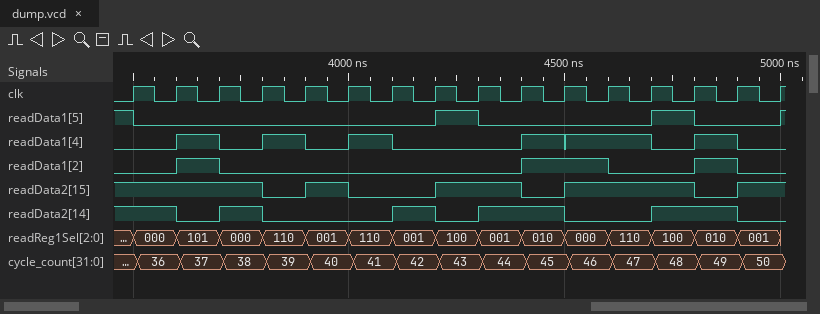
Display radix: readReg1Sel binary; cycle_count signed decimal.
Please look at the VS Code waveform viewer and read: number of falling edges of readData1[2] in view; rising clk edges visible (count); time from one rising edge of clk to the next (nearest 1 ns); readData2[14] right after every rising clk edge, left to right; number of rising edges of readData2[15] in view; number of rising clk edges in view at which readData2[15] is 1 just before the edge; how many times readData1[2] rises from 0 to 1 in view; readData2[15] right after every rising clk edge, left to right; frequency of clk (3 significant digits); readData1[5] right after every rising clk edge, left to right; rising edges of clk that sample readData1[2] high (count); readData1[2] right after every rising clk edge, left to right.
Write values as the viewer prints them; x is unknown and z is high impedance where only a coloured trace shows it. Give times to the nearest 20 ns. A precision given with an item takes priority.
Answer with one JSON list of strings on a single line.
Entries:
["3", "16", "100 ns", "1 0 1 0 0 0 1 0 1 1 0 0 1 1 0 0", "4", "11", "3", "1 1 1 0 1 0 0 1 1 0 1 1 1 0 1 1", "10.0 MHz", "0 0 0 0 0 0 0 1 0 0 0 0 1 0 0 1", "4", "0 1 0 0 0 0 0 0 0 1 1 0 0 1 0 0"]
